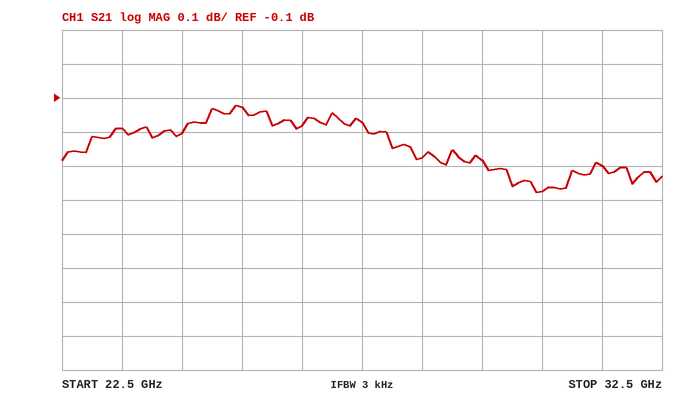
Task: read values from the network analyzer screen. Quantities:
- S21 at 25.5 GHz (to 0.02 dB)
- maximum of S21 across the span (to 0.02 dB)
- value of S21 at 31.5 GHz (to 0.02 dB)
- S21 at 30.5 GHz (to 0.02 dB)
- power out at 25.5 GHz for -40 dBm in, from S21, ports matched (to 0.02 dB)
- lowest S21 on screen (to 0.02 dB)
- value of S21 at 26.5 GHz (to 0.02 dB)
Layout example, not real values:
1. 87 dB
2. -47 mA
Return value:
1. -0.12 dB
2. -0.12 dB
3. -0.30 dB
4. -0.38 dB
5. -40.12 dBm
6. -0.38 dB
7. -0.18 dB
